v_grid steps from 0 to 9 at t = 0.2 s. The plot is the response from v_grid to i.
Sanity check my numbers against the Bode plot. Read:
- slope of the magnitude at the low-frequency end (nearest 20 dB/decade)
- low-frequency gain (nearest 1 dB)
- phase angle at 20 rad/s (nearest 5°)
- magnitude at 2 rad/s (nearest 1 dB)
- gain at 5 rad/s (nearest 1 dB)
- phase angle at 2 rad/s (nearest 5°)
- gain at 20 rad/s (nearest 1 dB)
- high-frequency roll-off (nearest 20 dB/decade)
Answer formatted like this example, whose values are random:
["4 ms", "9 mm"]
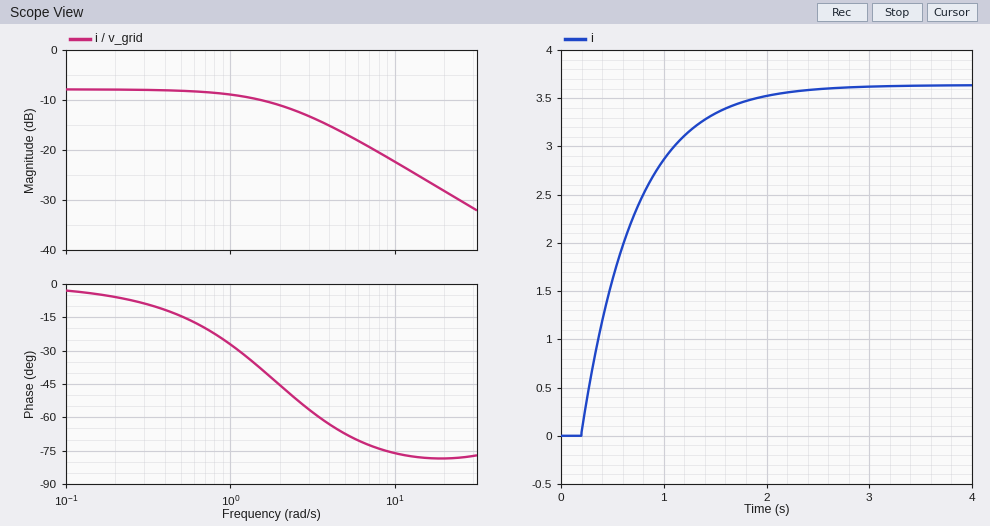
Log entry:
["0 dB/decade", "-8 dB", "-80°", "-11 dB", "-17 dB", "-45°", "-28 dB", "-20 dB/decade"]
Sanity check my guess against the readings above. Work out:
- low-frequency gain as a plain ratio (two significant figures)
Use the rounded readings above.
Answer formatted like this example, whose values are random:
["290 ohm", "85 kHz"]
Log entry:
["0.40"]
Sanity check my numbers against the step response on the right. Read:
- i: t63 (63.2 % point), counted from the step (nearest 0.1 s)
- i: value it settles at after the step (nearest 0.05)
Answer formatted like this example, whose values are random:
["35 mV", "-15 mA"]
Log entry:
["0.5 s", "3.65"]
